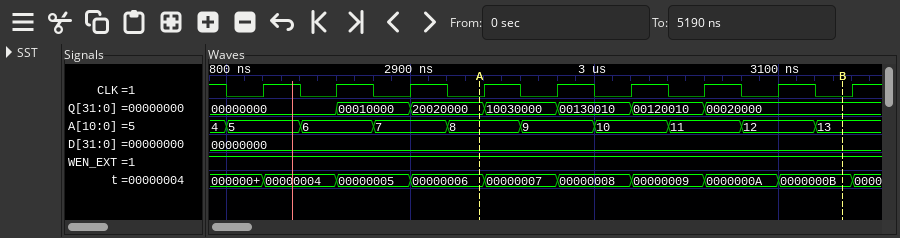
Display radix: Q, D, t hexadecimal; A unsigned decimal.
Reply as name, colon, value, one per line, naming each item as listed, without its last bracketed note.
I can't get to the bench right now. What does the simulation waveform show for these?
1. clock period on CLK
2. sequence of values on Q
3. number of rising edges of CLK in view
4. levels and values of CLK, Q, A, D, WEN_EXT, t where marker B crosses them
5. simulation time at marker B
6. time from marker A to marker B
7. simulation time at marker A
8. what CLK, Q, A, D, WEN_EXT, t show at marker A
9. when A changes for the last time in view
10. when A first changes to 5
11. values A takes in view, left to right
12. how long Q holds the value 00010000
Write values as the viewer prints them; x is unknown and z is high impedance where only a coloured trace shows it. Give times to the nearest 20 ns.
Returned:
clock period on CLK: 40 ns
sequence of values on Q: 00000000, 00010000, 20020000, 10030000, 00130010, 00120010, 00020000
number of rising edges of CLK in view: 9
levels and values of CLK, Q, A, D, WEN_EXT, t where marker B crosses them: CLK=0, Q=00020000, A=13, D=00000000, WEN_EXT=1, t=0000000B
simulation time at marker B: 3140 ns
time from marker A to marker B: 200 ns
simulation time at marker A: 2940 ns
what CLK, Q, A, D, WEN_EXT, t show at marker A: CLK=0, Q=20020000, A=8, D=00000000, WEN_EXT=1, t=00000006
when A changes for the last time in view: 3120 ns
when A first changes to 5: 2800 ns
values A takes in view, left to right: 4, 5, 6, 7, 8, 9, 10, 11, 12, 13
how long Q holds the value 00010000: 40 ns
